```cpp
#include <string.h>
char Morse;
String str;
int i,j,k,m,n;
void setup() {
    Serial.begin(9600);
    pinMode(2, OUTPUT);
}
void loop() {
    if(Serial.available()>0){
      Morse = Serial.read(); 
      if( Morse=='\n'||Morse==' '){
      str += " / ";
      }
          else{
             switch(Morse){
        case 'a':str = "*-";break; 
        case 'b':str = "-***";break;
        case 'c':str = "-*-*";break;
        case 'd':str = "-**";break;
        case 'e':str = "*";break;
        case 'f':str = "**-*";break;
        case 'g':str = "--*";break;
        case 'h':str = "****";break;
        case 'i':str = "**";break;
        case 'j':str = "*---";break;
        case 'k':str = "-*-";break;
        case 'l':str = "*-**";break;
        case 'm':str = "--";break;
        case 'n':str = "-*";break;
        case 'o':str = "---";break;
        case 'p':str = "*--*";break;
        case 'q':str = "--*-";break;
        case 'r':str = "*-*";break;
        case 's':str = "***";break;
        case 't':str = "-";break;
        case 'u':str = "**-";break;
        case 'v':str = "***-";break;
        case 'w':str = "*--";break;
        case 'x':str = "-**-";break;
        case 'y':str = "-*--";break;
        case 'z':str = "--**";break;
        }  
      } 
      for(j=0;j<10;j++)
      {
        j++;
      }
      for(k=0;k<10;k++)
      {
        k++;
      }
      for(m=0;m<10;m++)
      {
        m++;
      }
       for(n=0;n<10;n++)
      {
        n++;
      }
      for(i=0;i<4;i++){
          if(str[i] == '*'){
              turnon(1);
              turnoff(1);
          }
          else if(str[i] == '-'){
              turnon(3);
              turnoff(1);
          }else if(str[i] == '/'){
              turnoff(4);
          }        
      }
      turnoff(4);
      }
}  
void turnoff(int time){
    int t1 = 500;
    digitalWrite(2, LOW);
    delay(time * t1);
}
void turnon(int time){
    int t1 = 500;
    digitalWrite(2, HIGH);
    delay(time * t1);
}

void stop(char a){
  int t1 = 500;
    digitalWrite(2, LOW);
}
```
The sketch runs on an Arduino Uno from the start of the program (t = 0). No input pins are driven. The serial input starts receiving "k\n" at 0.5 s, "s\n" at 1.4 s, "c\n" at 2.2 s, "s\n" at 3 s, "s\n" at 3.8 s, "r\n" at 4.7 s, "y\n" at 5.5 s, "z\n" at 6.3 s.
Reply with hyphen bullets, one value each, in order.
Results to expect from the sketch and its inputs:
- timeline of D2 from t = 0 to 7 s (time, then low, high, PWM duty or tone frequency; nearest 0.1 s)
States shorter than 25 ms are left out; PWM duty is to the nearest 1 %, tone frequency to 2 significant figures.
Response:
- 0 s low; 0.5 s high; 2 s low; 2.5 s high; 3 s low; 3.5 s high; 5 s low
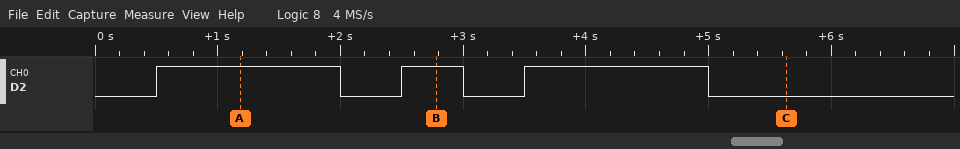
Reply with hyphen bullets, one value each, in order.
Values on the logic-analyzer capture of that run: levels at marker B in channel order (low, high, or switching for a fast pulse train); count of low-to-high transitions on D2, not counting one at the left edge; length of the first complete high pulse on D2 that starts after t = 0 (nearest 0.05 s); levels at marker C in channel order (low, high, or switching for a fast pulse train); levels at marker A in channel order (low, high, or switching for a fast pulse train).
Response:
- D2 high
- 3
- 1.50 s
- D2 low
- D2 high
